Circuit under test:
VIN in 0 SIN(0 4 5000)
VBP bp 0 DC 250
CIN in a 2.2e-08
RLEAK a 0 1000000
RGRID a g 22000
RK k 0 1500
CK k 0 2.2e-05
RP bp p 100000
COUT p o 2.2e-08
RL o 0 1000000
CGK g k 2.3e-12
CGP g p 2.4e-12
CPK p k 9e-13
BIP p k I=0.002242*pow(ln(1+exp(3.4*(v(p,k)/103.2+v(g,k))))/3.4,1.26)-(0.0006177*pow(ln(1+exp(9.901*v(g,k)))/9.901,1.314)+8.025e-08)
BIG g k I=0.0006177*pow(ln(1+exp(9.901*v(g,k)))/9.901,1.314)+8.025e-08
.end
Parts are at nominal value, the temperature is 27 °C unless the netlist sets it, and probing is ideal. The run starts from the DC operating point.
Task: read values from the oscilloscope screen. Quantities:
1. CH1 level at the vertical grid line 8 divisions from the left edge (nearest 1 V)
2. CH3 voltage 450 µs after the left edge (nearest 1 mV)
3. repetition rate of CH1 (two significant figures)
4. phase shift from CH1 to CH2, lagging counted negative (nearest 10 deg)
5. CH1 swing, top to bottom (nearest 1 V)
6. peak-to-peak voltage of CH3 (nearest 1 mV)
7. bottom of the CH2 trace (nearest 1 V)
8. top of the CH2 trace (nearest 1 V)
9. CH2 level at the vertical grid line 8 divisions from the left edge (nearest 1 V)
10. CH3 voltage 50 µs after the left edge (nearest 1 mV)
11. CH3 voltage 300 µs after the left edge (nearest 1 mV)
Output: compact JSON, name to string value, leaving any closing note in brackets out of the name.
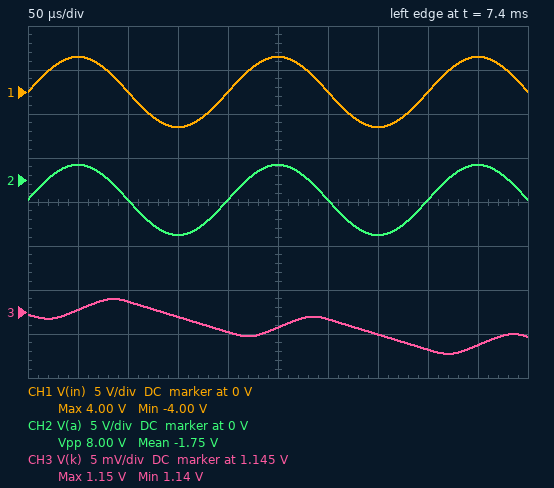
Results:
{"CH1 level at the vertical grid line 8 divisions from the left edge": "0 V", "CH3 voltage 450 µs after the left edge": "1.141 V", "repetition rate of CH1": "5.0 kHz", "phase shift from CH1 to CH2, lagging counted negative": "0 deg", "CH1 swing, top to bottom": "8 V", "peak-to-peak voltage of CH3": "6 mV", "bottom of the CH2 trace": "-6 V", "top of the CH2 trace": "2 V", "CH2 level at the vertical grid line 8 divisions from the left edge": "-2 V", "CH3 voltage 50 µs after the left edge": "1.145 V", "CH3 voltage 300 µs after the left edge": "1.144 V"}
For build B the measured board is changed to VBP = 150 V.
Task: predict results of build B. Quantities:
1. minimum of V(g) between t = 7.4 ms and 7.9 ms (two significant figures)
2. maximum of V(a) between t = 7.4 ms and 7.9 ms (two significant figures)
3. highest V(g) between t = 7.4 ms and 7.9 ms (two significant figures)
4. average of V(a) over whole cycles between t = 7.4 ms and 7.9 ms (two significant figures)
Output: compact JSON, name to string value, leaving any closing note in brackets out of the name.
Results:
{"minimum of V(g) between t = 7.4 ms and 7.9 ms": "-6.7 V", "maximum of V(a) between t = 7.4 ms and 7.9 ms": "1.3 V", "highest V(g) between t = 7.4 ms and 7.9 ms": "730 mV", "average of V(a) over whole cycles between t = 7.4 ms and 7.9 ms": "-2.7 V"}
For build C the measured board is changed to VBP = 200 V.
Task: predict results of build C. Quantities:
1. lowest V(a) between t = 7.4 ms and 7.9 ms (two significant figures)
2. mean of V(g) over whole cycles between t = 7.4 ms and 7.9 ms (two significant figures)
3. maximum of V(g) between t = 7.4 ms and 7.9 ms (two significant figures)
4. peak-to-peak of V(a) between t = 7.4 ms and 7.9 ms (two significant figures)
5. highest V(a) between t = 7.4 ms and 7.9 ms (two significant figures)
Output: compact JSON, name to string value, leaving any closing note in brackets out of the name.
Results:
{"lowest V(a) between t = 7.4 ms and 7.9 ms": "-6.5 V", "mean of V(g) over whole cycles between t = 7.4 ms and 7.9 ms": "-2.5 V", "maximum of V(g) between t = 7.4 ms and 7.9 ms": "950 mV", "peak-to-peak of V(a) between t = 7.4 ms and 7.9 ms": "8.0 V", "highest V(a) between t = 7.4 ms and 7.9 ms": "1.5 V"}
